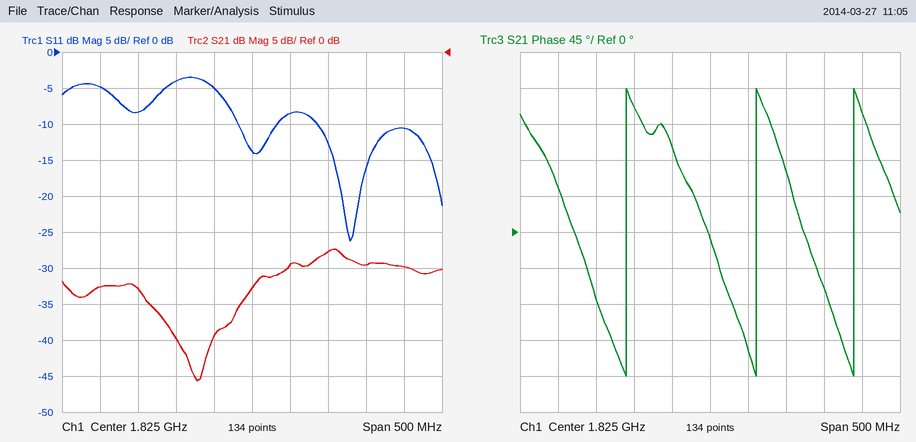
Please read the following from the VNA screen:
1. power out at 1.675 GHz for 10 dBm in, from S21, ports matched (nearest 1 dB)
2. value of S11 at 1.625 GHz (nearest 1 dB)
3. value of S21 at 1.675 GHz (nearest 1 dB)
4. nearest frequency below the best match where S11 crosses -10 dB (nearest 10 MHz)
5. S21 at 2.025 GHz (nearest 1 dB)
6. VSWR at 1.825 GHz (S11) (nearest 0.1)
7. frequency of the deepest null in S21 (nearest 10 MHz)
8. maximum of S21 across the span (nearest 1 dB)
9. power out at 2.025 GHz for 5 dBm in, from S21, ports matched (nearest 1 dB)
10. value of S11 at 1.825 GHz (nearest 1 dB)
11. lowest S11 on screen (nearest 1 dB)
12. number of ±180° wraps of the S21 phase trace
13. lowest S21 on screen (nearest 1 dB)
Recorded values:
-23 dBm
-5 dB
-33 dB
1.91 GHz
-30 dB
1.5
1.75 GHz
-27 dB
-25 dBm
-14 dB
-26 dB
3
-46 dB
